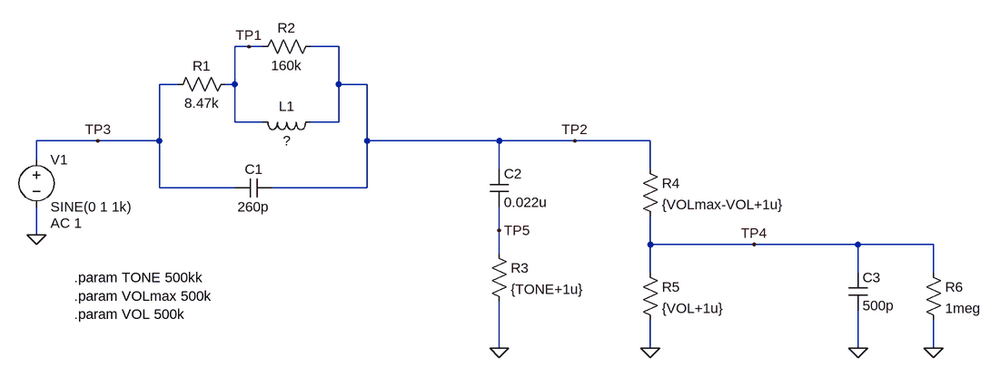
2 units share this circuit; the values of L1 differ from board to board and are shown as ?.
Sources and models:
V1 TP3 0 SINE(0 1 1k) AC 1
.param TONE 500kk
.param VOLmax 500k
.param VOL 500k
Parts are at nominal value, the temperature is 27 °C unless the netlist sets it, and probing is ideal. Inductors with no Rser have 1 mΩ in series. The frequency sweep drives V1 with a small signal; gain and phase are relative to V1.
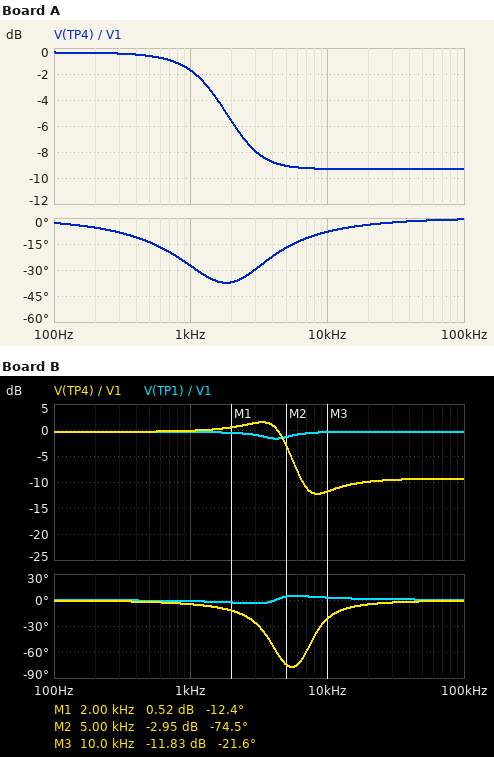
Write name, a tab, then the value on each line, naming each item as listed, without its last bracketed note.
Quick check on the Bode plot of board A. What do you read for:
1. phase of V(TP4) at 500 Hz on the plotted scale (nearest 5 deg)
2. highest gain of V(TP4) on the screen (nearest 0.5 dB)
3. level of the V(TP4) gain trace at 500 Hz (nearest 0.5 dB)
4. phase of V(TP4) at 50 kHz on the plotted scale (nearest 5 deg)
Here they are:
phase of V(TP4) at 500 Hz on the plotted scale	-15 deg
highest gain of V(TP4) on the screen	-0.5 dB
level of the V(TP4) gain trace at 500 Hz	-0.5 dB
phase of V(TP4) at 50 kHz on the plotted scale	0 deg
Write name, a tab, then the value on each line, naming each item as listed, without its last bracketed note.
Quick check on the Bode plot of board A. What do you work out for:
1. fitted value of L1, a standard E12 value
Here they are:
fitted value of L1, a standard E12 value	15 H
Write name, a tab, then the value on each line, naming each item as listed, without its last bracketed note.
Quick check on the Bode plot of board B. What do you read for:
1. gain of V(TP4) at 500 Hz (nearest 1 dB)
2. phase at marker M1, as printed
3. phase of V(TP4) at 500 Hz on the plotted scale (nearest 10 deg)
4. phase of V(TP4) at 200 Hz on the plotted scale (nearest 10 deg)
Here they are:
gain of V(TP4) at 500 Hz	0 dB
phase at marker M1, as printed	-12.4 deg
phase of V(TP4) at 500 Hz on the plotted scale	0 deg
phase of V(TP4) at 200 Hz on the plotted scale	0 deg
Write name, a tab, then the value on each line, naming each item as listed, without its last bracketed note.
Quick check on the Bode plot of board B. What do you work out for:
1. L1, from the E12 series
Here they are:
L1, from the E12 series	1.8 H
